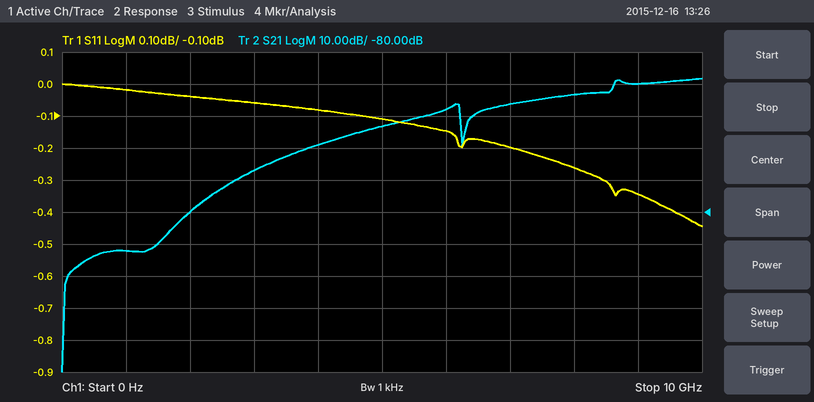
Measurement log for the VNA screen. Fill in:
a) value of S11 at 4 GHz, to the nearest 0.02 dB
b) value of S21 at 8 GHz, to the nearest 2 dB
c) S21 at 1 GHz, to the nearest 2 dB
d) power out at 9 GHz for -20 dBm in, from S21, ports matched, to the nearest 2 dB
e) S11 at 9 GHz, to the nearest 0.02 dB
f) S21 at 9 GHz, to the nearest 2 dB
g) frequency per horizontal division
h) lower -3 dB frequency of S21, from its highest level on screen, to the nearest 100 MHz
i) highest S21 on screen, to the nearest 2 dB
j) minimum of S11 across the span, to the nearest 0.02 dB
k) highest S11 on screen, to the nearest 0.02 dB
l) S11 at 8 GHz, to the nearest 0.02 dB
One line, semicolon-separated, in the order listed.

-0.08 dB; -44 dB; -92 dB; -60 dBm; -0.34 dB; -40 dB; 1 GHz; 8.6 GHz; -38 dB; -0.44 dB; 0.00 dB; -0.26 dB
